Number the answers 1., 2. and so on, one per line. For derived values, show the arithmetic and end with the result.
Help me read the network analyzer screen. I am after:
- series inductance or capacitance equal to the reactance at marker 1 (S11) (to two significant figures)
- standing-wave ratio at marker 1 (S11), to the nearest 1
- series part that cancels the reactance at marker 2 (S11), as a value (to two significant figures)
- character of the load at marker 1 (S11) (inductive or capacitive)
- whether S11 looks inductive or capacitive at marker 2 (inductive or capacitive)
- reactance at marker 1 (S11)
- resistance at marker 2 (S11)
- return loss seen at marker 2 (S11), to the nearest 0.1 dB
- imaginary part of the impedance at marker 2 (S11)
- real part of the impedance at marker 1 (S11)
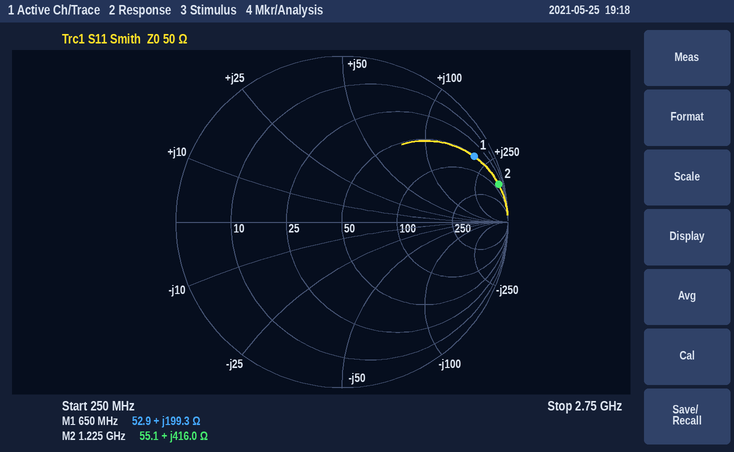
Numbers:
1. L = 199.3 Ω/(2π × 650 MHz) ≈ 49 nH
2. 17
3. C = 1/(2π × 1.225 GHz × 416 Ω) ≈ 312 fF, so 310 fF to two significant figures
4. inductive
5. inductive
6. +199.3 Ω
7. 55.1 Ω
8. 0.3 dB
9. +416.0 Ω
10. 52.9 Ω
